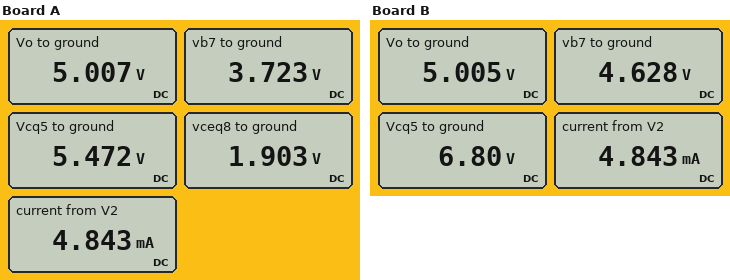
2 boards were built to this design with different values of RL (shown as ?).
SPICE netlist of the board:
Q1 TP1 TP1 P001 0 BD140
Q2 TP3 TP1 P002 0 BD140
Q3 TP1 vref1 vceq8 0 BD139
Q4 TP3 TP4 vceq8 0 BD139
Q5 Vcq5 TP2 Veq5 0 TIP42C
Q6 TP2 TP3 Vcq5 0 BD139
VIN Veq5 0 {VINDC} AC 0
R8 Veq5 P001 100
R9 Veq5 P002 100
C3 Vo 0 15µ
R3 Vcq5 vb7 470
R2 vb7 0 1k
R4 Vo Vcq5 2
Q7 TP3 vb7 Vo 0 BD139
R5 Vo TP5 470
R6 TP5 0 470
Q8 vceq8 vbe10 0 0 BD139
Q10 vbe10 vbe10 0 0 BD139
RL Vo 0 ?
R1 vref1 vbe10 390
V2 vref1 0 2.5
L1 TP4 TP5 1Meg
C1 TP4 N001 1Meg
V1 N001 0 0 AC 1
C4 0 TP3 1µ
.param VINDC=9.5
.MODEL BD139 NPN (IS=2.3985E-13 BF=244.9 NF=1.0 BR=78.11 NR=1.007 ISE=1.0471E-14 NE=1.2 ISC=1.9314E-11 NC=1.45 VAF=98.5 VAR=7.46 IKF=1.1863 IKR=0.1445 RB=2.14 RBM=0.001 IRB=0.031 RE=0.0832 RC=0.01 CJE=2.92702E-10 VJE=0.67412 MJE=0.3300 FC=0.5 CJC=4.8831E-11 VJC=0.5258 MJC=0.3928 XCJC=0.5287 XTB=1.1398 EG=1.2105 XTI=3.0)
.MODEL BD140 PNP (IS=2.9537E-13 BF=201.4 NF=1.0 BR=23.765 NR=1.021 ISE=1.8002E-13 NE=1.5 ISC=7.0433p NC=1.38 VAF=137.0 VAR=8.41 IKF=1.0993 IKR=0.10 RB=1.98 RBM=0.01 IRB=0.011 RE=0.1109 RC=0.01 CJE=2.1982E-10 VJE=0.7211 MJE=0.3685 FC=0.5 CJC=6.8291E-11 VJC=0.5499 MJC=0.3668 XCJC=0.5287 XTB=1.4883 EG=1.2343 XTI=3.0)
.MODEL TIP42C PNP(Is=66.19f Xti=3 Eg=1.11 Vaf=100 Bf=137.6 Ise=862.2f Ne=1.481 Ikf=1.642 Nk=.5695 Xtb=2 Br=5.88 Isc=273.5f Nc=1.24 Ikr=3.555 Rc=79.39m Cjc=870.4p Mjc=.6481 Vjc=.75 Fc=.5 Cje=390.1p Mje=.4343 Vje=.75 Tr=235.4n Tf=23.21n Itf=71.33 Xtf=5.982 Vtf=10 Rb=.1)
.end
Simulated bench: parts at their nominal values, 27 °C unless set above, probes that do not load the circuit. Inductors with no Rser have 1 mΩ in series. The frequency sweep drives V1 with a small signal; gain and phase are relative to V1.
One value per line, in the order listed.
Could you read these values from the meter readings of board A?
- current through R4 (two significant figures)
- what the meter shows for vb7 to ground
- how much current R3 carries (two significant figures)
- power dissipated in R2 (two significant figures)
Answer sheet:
230 mA
3.723 V
3.7 mA
14 mW
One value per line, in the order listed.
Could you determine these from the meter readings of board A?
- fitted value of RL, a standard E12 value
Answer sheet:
22 Ω
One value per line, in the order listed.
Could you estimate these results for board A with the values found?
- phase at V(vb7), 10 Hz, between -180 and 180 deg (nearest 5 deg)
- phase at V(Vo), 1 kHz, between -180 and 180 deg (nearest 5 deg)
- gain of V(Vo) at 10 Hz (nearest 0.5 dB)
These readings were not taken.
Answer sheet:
115 deg
80 deg
61.5 dB
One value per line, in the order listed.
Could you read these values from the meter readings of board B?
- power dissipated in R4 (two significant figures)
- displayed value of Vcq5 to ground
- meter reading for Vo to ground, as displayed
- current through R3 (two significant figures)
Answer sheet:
1.6 W
6.80 V
5.005 V
4.6 mA
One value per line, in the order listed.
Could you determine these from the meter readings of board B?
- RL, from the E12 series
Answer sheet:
5.6 Ω
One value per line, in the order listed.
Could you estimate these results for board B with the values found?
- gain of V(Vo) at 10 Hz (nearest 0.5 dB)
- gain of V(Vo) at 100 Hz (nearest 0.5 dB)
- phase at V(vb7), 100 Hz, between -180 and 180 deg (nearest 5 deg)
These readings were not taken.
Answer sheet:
59.0 dB
40.5 dB
95 deg
